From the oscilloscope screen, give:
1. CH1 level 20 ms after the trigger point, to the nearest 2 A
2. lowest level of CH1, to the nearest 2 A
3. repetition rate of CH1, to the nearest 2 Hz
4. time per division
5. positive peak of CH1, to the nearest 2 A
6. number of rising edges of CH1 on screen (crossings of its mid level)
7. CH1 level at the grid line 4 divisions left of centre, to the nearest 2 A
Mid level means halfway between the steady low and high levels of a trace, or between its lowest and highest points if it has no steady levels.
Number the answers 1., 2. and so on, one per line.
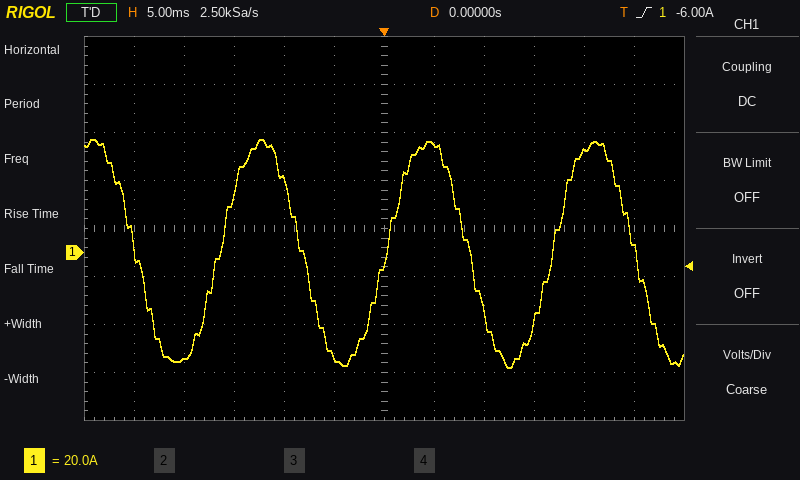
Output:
1. 42 A
2. -48 A
3. 60 Hz
4. 5 ms
5. 48 A
6. 3
7. -44 A
